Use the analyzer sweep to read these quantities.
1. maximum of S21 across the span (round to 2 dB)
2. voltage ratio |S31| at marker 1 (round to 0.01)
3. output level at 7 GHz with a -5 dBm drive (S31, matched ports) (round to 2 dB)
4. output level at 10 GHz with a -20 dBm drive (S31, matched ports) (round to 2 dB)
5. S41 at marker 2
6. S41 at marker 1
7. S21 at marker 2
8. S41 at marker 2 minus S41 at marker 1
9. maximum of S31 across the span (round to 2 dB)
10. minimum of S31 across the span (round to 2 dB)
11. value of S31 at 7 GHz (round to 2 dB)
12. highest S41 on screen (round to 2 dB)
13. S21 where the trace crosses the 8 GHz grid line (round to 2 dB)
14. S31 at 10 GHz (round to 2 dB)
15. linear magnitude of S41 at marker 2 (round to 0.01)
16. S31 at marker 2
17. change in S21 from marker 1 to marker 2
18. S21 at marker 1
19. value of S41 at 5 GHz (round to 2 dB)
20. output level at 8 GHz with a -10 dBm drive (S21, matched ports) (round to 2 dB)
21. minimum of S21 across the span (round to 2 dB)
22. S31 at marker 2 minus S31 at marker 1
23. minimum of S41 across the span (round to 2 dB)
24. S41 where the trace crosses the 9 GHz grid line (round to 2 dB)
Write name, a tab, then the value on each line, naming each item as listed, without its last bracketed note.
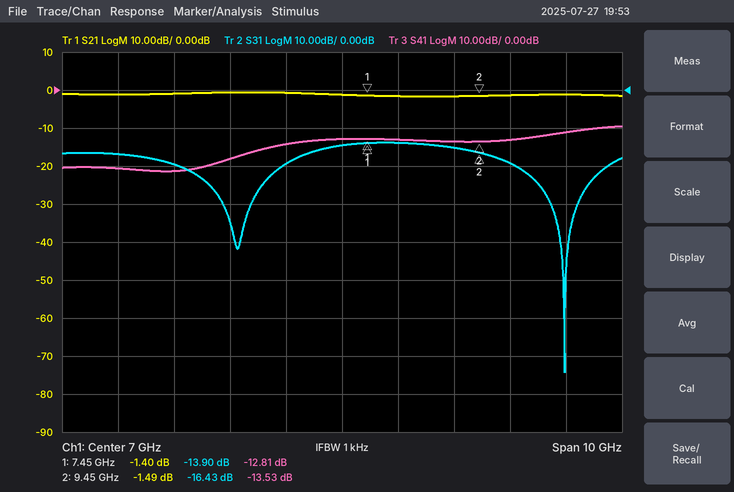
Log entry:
maximum of S21 across the span	0 dB
voltage ratio |S31| at marker 1	0.20
output level at 7 GHz with a -5 dBm drive (S31, matched ports)	-20 dBm
output level at 10 GHz with a -20 dBm drive (S31, matched ports)	-40 dBm
S41 at marker 2	-13.53 dB
S41 at marker 1	-12.81 dB
S21 at marker 2	-1.49 dB
S41 at marker 2 minus S41 at marker 1	-0.72 dB
maximum of S31 across the span	-14 dB
minimum of S31 across the span	-74 dB
value of S31 at 7 GHz	-14 dB
highest S41 on screen	-10 dB
S21 where the trace crosses the 8 GHz grid line	-2 dB
S31 at 10 GHz	-20 dB
linear magnitude of S41 at marker 2	0.21
S31 at marker 2	-16.43 dB
change in S21 from marker 1 to marker 2	-0.09 dB
S21 at marker 1	-1.40 dB
value of S41 at 5 GHz	-18 dB
output level at 8 GHz with a -10 dBm drive (S21, matched ports)	-12 dBm
minimum of S21 across the span	-2 dB
S31 at marker 2 minus S31 at marker 1	-2.53 dB
minimum of S41 across the span	-22 dB
S41 where the trace crosses the 9 GHz grid line	-14 dB
